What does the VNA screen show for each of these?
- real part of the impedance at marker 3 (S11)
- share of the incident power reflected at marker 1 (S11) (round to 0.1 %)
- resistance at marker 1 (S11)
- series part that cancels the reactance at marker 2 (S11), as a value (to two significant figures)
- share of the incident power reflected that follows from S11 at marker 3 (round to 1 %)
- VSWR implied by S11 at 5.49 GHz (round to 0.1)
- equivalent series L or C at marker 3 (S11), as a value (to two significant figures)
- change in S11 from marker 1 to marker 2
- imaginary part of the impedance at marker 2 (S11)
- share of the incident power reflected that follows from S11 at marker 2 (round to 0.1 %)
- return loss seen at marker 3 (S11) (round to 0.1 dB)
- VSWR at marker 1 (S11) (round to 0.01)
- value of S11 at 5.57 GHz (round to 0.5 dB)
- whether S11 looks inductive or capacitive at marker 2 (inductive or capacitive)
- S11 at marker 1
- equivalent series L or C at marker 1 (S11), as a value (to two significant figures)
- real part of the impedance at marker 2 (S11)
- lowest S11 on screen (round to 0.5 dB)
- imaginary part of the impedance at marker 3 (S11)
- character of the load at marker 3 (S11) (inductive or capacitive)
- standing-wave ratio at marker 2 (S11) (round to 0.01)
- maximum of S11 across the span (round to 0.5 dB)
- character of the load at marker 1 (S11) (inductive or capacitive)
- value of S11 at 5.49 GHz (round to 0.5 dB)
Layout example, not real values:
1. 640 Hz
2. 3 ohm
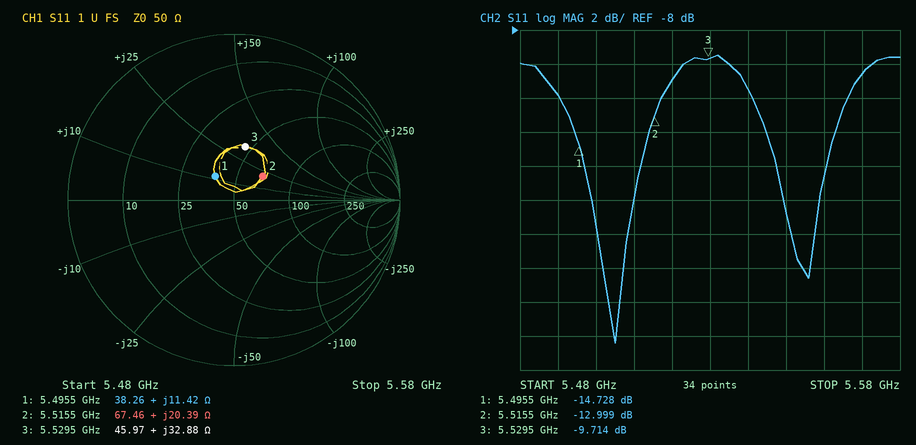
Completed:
1. 45.97 Ω
2. 3.4 %
3. 38.26 Ω
4. 1.4 pF
5. 11 %
6. 1.7
7. 950 pH
8. 1.729 dB
9. +20.39 Ω
10. 5.0 %
11. 9.7 dB
12. 1.45
13. -10.5 dB
14. inductive
15. -14.728 dB
16. 330 pH
17. 67.46 Ω
18. -26.5 dB
19. +32.88 Ω
20. inductive
21. 1.58
22. -9.5 dB
23. inductive
24. -12.0 dB
